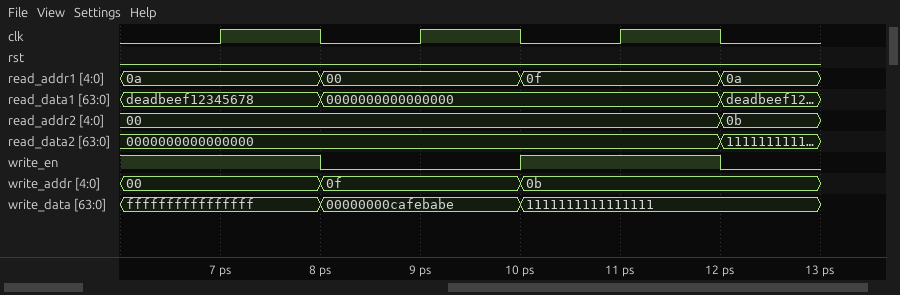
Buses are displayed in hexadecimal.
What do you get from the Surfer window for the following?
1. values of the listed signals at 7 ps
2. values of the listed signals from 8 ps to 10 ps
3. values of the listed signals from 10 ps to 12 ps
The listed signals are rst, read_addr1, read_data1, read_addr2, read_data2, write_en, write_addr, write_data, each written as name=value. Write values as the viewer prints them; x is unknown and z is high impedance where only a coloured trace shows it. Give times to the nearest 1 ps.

rst=0, read_addr1=0a, read_data1=deadbeef12345678, read_addr2=00, read_data2=0000000000000000, write_en=1, write_addr=00, write_data=ffffffffffffffff
rst=0, read_addr1=00, read_data1=0000000000000000, read_addr2=00, read_data2=0000000000000000, write_en=0, write_addr=0f, write_data=00000000cafebabe
rst=0, read_addr1=0f, read_data1=0000000000000000, read_addr2=00, read_data2=0000000000000000, write_en=1, write_addr=0b, write_data=1111111111111111
